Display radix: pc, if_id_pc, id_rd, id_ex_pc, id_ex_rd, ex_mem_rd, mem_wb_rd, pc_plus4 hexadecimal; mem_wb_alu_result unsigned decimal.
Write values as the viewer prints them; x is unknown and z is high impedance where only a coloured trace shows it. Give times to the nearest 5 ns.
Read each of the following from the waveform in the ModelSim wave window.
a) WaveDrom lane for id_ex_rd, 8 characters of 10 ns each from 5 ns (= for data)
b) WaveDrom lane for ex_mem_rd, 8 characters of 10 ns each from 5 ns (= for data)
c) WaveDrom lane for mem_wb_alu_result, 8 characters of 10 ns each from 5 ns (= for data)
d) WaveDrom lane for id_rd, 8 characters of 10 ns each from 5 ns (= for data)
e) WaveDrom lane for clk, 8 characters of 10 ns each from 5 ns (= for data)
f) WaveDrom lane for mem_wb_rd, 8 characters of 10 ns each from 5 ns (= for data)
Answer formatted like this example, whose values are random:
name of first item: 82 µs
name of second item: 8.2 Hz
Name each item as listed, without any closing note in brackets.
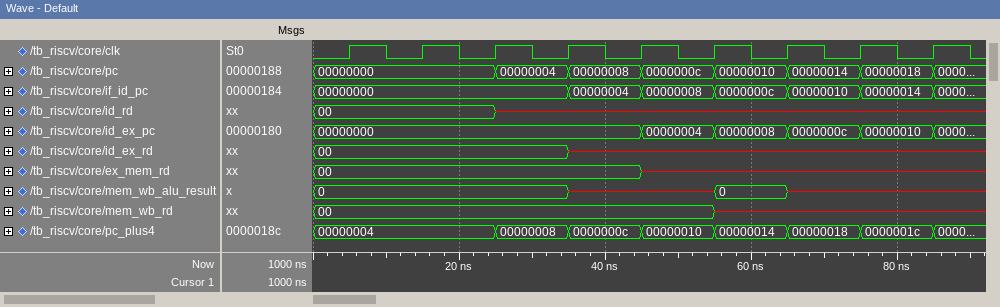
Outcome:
WaveDrom lane for id_ex_rd, 8 characters of 10 ns each from 5 ns: {name: 'id_ex_rd', wave: '=..x....', data: '00'}
WaveDrom lane for ex_mem_rd, 8 characters of 10 ns each from 5 ns: {name: 'ex_mem_rd', wave: '=...x...', data: '00'}
WaveDrom lane for mem_wb_alu_result, 8 characters of 10 ns each from 5 ns: {name: 'mem_wb_alu_result', wave: '=..x.=x.', data: '0 0'}
WaveDrom lane for id_rd, 8 characters of 10 ns each from 5 ns: {name: 'id_rd', wave: '=.x.....', data: '00'}
WaveDrom lane for clk, 8 characters of 10 ns each from 5 ns: {name: 'clk', wave: 'p.......'}
WaveDrom lane for mem_wb_rd, 8 characters of 10 ns each from 5 ns: {name: 'mem_wb_rd', wave: '=....x..', data: '00'}
